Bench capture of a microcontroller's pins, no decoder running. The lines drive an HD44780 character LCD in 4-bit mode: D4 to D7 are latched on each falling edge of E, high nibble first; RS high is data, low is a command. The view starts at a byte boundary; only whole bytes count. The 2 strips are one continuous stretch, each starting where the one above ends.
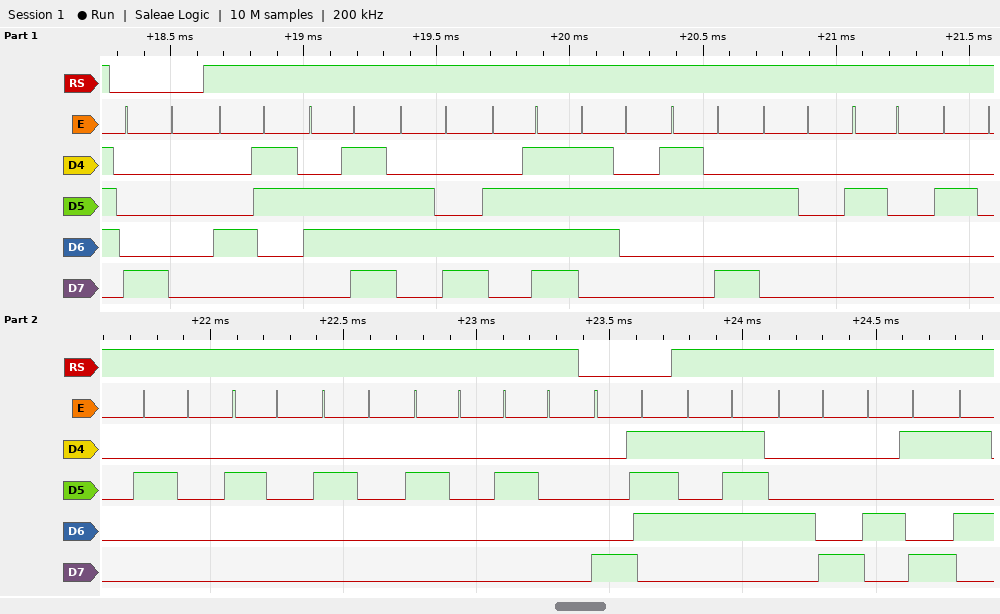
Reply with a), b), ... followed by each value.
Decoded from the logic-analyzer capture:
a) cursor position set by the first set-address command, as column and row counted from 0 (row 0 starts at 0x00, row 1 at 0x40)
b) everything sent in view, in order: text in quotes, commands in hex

a) column 0, row 0
b) 0x80 "Color:        " 0x87 "WHI"
